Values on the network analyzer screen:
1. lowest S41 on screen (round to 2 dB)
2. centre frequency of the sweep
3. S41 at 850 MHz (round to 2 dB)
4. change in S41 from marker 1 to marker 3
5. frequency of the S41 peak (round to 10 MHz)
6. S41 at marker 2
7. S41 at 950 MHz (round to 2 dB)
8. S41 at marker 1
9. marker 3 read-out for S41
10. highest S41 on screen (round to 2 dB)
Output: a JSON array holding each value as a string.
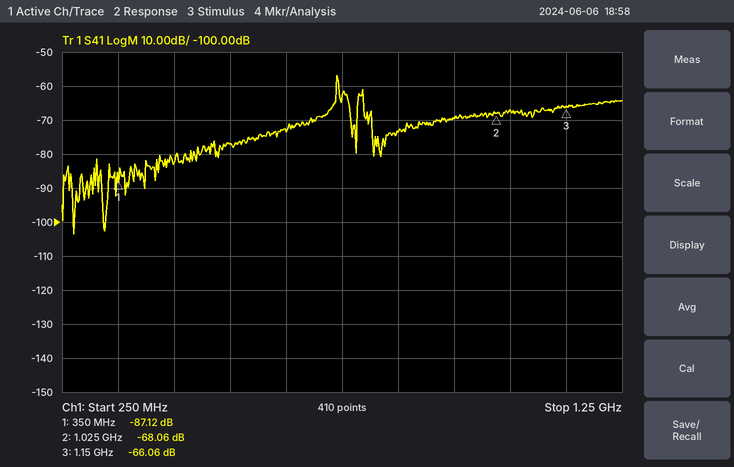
["-104 dB", "750 MHz", "-74 dB", "21.06 dB", "740 MHz", "-68.06 dB", "-70 dB", "-87.12 dB", "-66.06 dB", "-56 dB"]
